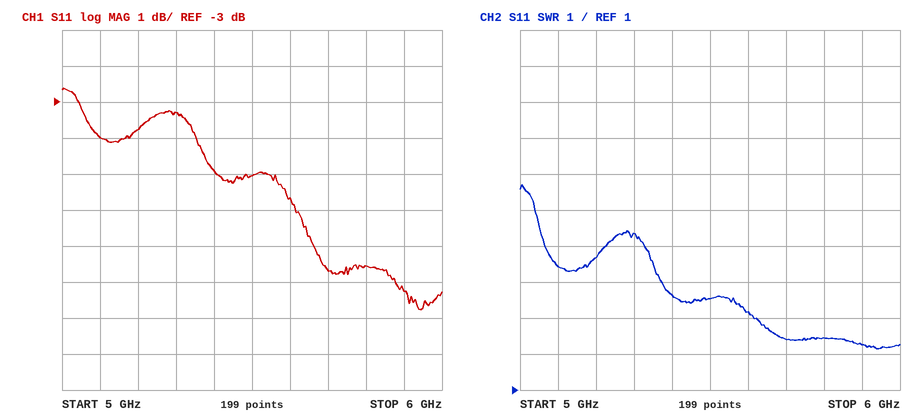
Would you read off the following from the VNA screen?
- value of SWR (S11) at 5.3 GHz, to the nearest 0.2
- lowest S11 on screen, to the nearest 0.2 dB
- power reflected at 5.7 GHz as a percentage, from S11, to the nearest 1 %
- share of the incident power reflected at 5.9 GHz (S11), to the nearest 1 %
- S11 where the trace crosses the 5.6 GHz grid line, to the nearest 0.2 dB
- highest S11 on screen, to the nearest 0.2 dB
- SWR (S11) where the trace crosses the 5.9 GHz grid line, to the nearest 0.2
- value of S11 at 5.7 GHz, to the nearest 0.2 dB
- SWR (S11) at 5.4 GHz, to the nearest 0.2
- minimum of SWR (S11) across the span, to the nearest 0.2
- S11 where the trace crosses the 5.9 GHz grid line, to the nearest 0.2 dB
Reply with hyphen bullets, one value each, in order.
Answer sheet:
- 5.4
- -8.8 dB
- 17 %
- 15 %
- -5.6 dB
- -2.6 dB
- 2.2
- -7.6 dB
- 3.6
- 2.2
- -8.2 dB
